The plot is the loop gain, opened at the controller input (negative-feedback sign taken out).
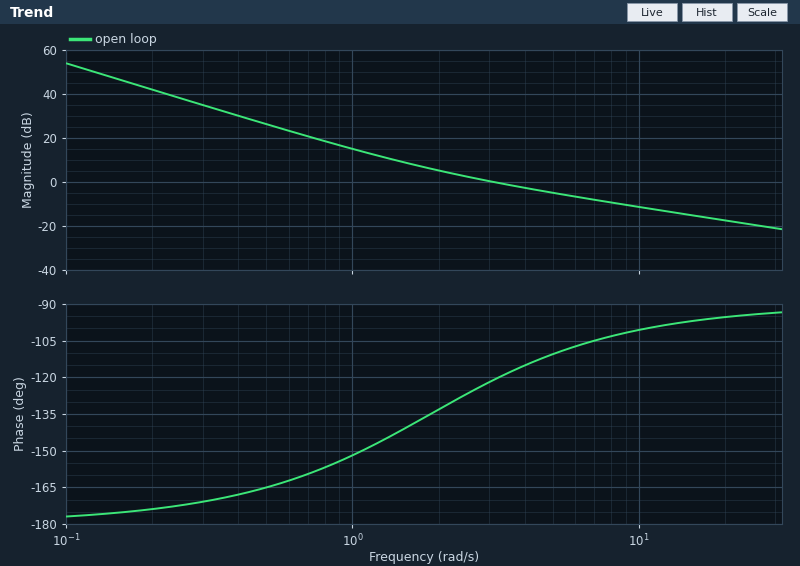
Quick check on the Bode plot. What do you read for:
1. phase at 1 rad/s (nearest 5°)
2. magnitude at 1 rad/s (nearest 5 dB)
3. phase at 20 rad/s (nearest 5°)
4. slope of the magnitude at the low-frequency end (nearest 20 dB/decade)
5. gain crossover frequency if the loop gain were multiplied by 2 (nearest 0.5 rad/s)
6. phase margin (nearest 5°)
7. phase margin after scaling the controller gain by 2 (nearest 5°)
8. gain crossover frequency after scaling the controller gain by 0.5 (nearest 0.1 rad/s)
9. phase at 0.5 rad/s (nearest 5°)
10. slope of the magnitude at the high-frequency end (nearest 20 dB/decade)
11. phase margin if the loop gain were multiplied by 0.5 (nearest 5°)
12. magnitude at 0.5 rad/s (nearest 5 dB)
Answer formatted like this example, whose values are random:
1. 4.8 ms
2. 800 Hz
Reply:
1. -150°
2. 15 dB
3. -95°
4. -40 dB/decade
5. 5.5 rad/s
6. 60°
7. 70°
8. 1.9 rad/s
9. -165°
10. -20 dB/decade
11. 45°
12. 25 dB
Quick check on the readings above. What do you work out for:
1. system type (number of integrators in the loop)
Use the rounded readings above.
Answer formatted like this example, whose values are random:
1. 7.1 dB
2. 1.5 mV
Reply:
1. 2
